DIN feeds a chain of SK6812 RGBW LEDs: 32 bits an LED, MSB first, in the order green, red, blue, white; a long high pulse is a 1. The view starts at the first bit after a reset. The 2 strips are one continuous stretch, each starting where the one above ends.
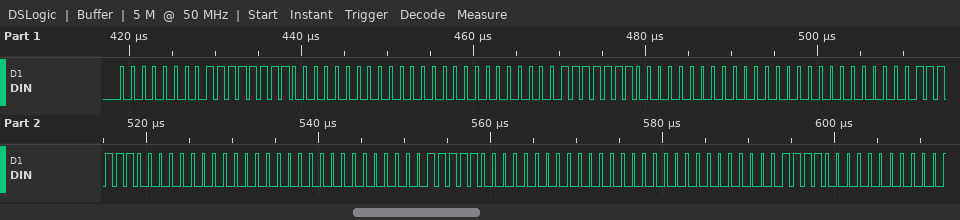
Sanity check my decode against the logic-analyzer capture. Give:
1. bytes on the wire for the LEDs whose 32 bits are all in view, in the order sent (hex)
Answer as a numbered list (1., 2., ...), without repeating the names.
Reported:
1. 00 FF 00 00 00 7F 00 00 00 3F 00 00 00 1F 00 00
